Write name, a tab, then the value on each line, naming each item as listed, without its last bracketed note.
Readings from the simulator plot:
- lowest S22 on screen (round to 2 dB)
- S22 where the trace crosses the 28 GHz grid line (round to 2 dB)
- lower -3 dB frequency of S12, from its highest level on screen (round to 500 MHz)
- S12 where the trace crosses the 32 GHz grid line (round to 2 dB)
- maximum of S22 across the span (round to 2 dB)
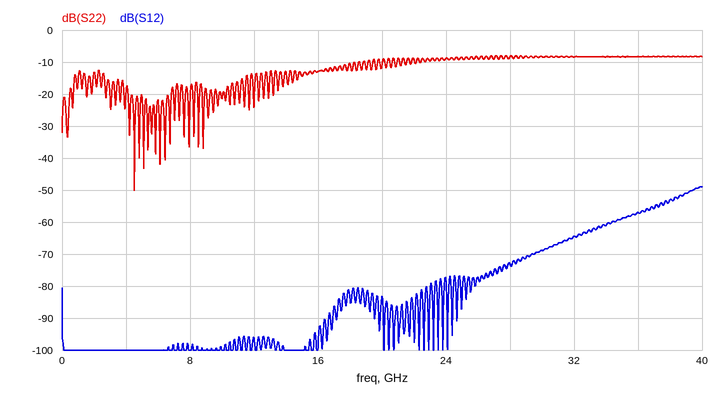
lowest S22 on screen	-50 dB
S22 where the trace crosses the 28 GHz grid line	-8 dB
lower -3 dB frequency of S12, from its highest level on screen	38.5 GHz
S12 where the trace crosses the 32 GHz grid line	-64 dB
maximum of S22 across the span	-8 dB
